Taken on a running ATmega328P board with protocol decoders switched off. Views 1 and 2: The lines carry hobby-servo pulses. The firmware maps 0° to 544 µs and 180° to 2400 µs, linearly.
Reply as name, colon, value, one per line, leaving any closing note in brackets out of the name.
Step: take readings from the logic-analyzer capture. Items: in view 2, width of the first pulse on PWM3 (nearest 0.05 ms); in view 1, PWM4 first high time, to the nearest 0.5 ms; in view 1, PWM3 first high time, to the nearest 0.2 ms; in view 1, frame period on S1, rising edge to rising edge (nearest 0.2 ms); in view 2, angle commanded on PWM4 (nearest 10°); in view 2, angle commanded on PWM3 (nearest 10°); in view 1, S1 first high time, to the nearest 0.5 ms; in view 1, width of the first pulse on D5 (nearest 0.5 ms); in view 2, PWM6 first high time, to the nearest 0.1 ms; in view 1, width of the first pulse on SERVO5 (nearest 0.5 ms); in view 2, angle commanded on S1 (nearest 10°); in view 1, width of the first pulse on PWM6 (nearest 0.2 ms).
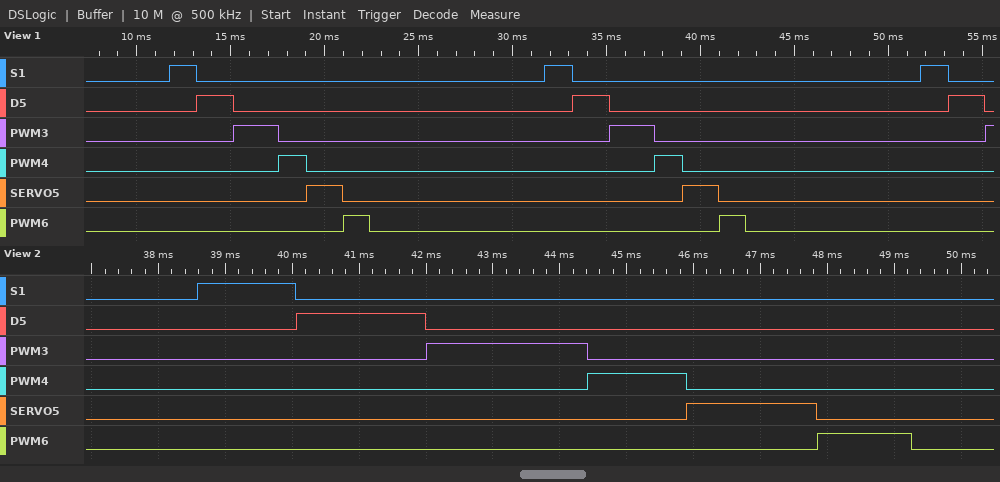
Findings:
in view 2, width of the first pulse on PWM3: 2.40 ms
in view 1, PWM4 first high time, to the nearest 0.5 ms: 1.5 ms
in view 1, PWM3 first high time, to the nearest 0.2 ms: 2.4 ms
in view 1, frame period on S1, rising edge to rising edge: 20.0 ms
in view 2, angle commanded on PWM4: 90°
in view 2, angle commanded on PWM3: 180°
in view 1, S1 first high time, to the nearest 0.5 ms: 1.5 ms
in view 1, width of the first pulse on D5: 2.0 ms
in view 2, PWM6 first high time, to the nearest 0.1 ms: 1.4 ms
in view 1, width of the first pulse on SERVO5: 2.0 ms
in view 2, angle commanded on S1: 90°
in view 1, width of the first pulse on PWM6: 1.4 ms
